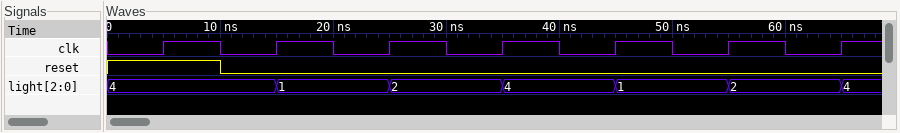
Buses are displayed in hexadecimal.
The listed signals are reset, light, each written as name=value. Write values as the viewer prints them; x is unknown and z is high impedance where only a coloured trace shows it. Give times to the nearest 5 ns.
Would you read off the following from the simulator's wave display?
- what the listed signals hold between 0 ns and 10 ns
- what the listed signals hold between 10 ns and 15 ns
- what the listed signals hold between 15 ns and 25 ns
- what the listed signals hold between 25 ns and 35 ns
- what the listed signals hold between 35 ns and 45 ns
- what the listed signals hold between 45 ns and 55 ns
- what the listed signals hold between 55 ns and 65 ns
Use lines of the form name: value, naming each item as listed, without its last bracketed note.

what the listed signals hold between 0 ns and 10 ns: reset=1, light=4
what the listed signals hold between 10 ns and 15 ns: reset=0, light=4
what the listed signals hold between 15 ns and 25 ns: reset=0, light=1
what the listed signals hold between 25 ns and 35 ns: reset=0, light=2
what the listed signals hold between 35 ns and 45 ns: reset=0, light=4
what the listed signals hold between 45 ns and 55 ns: reset=0, light=1
what the listed signals hold between 55 ns and 65 ns: reset=0, light=2
